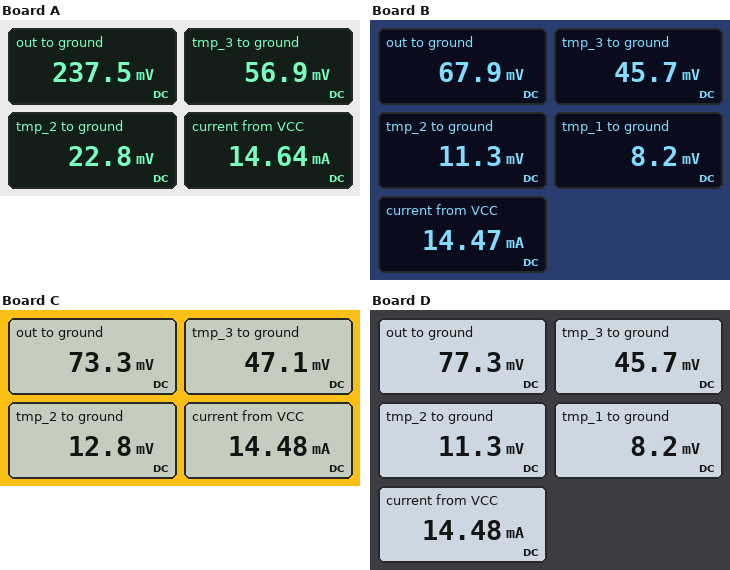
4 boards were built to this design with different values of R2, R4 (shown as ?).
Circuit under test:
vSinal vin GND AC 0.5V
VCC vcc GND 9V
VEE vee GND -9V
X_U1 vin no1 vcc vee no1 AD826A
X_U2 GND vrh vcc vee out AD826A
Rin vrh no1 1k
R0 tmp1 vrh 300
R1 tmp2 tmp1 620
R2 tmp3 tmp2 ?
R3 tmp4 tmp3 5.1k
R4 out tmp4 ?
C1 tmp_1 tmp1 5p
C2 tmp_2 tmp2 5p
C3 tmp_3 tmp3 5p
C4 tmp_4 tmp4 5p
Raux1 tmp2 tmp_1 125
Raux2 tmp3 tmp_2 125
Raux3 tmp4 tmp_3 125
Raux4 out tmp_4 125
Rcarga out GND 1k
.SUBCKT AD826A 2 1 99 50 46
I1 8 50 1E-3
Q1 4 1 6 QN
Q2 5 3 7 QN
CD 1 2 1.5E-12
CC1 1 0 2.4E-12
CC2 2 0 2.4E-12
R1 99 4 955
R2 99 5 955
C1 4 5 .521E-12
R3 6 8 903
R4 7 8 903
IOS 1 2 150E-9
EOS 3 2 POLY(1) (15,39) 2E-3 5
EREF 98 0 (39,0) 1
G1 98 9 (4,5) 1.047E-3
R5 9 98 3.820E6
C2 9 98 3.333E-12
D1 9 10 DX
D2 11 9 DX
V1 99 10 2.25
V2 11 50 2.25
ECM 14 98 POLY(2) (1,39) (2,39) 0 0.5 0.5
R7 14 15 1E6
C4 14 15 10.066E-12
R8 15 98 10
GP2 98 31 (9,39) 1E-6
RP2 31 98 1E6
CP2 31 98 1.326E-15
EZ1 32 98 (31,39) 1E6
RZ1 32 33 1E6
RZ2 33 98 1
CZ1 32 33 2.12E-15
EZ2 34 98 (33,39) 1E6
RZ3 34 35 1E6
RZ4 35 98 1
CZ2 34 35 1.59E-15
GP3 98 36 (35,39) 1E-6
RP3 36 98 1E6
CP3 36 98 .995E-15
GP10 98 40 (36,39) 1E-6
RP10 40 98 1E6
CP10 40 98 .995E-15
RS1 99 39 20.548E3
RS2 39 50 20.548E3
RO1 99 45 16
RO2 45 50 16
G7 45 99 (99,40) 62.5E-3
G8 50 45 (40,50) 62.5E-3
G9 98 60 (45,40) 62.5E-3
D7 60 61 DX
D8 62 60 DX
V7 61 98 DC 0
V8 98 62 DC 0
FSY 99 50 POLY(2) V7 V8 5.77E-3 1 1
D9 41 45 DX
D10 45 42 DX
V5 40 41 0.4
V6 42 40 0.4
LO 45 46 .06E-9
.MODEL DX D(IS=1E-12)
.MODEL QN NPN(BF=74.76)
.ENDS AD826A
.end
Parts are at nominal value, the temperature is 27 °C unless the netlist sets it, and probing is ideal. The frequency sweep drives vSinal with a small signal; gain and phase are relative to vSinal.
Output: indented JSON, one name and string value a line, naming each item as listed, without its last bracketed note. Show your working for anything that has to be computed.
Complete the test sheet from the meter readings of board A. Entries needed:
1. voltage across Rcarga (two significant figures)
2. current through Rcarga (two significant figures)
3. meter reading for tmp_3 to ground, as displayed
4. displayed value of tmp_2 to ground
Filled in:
{
  "voltage across Rcarga": "237.5 mV = 240 mV",
  "current through Rcarga": "(237.5 mV) / 1 kΩ = 240 µA",
  "meter reading for tmp_3 to ground, as displayed": "56.9 mV",
  "displayed value of tmp_2 to ground": "22.8 mV"
}
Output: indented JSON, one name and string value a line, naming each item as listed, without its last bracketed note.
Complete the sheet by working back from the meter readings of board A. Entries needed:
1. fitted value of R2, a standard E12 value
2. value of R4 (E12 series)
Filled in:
{
  "fitted value of R2, a standard E12 value": "2.2 kΩ",
  "value of R4": "27 kΩ"
}
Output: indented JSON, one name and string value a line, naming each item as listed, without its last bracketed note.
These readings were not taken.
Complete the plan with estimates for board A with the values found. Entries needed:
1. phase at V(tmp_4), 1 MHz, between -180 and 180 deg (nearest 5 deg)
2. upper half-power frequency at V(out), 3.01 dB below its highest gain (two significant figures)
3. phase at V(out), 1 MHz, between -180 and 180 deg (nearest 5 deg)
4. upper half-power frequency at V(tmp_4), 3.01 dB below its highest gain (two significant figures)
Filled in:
{
  "phase at V(tmp_4), 1 MHz, between -180 and 180 deg": "125 deg",
  "upper half-power frequency at V(out), 3.01 dB below its highest gain": "690 kHz",
  "phase at V(out), 1 MHz, between -180 and 180 deg": "125 deg",
  "upper half-power frequency at V(tmp_4), 3.01 dB below its highest gain": "690 kHz"
}
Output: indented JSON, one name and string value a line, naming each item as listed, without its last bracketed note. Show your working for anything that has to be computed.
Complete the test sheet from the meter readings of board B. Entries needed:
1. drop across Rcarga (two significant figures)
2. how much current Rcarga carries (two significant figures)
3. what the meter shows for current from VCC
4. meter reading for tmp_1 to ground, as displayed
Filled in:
{
  "drop across Rcarga": "67.9 mV = 68 mV",
  "how much current Rcarga carries": "(67.9 mV) / 1 kΩ = 68 µA",
  "what the meter shows for current from VCC": "14.47 mA",
  "meter reading for tmp_1 to ground, as displayed": "8.2 mV"
}
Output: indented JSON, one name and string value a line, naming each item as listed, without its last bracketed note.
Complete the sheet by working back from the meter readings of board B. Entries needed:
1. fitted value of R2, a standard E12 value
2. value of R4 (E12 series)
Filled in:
{
  "fitted value of R2, a standard E12 value": "470 Ω",
  "value of R4": "3.3 kΩ"
}
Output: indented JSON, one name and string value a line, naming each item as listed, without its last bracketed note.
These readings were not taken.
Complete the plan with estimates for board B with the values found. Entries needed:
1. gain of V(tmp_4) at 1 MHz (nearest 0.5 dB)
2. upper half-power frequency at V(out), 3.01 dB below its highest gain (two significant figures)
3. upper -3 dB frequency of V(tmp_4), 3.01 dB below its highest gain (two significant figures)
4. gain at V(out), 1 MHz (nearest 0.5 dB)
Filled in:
{
  "gain of V(tmp_4) at 1 MHz": "19.5 dB",
  "upper half-power frequency at V(out), 3.01 dB below its highest gain": "3.1 MHz",
  "upper -3 dB frequency of V(tmp_4), 3.01 dB below its highest gain": "3.1 MHz",
  "gain at V(out), 1 MHz": "19.5 dB"
}
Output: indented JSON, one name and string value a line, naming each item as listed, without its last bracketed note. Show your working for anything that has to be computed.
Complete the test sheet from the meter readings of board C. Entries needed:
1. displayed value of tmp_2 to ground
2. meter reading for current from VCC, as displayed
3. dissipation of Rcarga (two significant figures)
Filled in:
{
  "displayed value of tmp_2 to ground": "12.8 mV",
  "meter reading for current from VCC, as displayed": "14.48 mA",
  "dissipation of Rcarga": "(73.3 mV)^2 / 1 kΩ = 5.4 µW"
}
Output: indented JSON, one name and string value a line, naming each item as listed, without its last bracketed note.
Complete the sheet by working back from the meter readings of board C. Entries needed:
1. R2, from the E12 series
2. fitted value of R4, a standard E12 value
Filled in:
{
  "R2, from the E12 series": "680 Ω",
  "fitted value of R4, a standard E12 value": "3.9 kΩ"
}
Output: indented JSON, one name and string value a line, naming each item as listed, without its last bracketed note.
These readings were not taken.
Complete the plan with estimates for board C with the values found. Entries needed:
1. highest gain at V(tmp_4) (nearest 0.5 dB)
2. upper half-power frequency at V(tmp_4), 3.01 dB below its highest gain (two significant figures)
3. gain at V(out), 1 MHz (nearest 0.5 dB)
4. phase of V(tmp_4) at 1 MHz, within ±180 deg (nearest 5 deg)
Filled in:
{
  "highest gain at V(tmp_4)": "20.5 dB",
  "upper half-power frequency at V(tmp_4), 3.01 dB below its highest gain": "2.9 MHz",
  "gain at V(out), 1 MHz": "20.0 dB",
  "phase of V(tmp_4) at 1 MHz, within ±180 deg": "160 deg"
}
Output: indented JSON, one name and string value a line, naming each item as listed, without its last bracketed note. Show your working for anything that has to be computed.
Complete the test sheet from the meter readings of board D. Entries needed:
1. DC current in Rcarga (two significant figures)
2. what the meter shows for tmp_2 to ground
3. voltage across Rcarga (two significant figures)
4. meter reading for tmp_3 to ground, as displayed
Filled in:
{
  "DC current in Rcarga": "(77.3 mV) / 1 kΩ = 77 µA",
  "what the meter shows for tmp_2 to ground": "11.3 mV",
  "voltage across Rcarga": "77.3 mV = 77 mV",
  "meter reading for tmp_3 to ground, as displayed": "45.7 mV"
}
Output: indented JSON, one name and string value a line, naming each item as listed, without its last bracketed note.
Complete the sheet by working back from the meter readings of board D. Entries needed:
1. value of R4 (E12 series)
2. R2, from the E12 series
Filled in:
{
  "value of R4": "4.7 kΩ",
  "R2, from the E12 series": "470 Ω"
}
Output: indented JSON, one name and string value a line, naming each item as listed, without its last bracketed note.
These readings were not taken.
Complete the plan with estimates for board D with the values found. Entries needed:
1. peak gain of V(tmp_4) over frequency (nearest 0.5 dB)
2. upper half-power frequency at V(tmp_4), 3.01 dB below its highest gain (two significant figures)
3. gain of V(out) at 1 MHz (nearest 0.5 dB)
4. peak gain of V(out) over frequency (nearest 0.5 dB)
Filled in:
{
  "peak gain of V(tmp_4) over frequency": "21.0 dB",
  "upper half-power frequency at V(tmp_4), 3.01 dB below its highest gain": "2.7 MHz",
  "gain of V(out) at 1 MHz": "20.5 dB",
  "peak gain of V(out) over frequency": "21.0 dB"
}
